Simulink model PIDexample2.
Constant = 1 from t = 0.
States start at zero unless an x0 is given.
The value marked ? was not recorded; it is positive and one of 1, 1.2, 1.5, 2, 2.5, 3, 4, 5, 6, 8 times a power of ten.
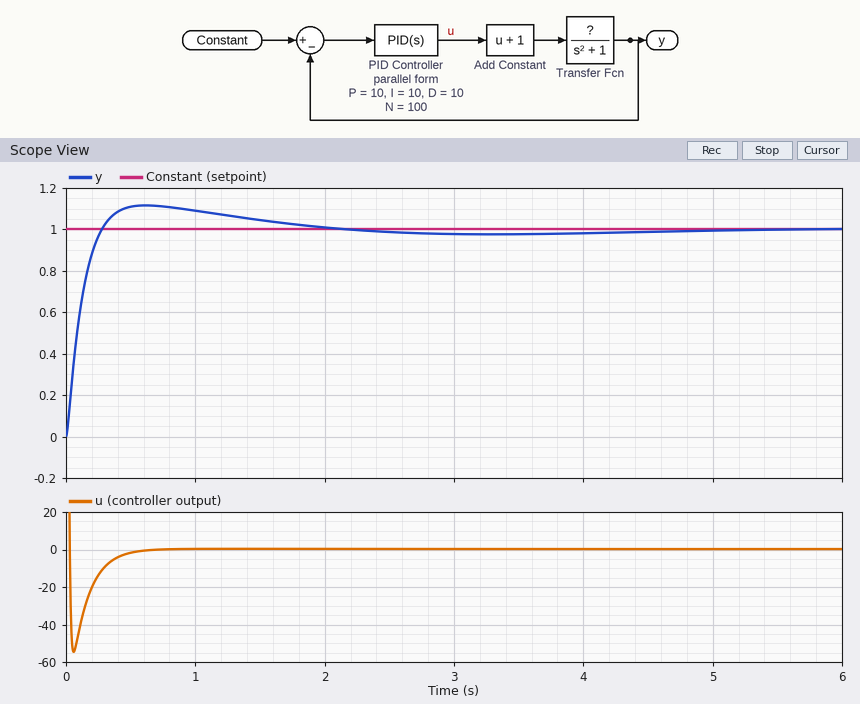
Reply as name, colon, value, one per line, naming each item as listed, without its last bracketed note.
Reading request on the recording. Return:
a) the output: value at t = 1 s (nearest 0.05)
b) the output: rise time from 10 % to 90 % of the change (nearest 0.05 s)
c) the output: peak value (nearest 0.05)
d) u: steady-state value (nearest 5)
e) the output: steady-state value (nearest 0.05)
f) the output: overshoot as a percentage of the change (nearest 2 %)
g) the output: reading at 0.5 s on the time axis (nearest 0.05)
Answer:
the output: value at t = 1 s: 1.10
the output: rise time from 10 % to 90 % of the change: 0.20 s
the output: peak value: 1.10
u: steady-state value: 0
the output: steady-state value: 1.00
the output: overshoot as a percentage of the change: 12 %
the output: reading at 0.5 s on the time axis: 1.10
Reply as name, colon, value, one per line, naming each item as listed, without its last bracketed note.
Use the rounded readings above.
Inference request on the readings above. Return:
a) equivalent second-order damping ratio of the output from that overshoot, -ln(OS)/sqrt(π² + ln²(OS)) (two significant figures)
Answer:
equivalent second-order damping ratio of the output from that overshoot, -ln(OS)/sqrt(π² + ln²(OS)): 0.56
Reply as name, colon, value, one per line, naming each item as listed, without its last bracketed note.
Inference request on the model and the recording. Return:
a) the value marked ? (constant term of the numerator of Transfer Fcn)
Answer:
the value marked ?: 0.8
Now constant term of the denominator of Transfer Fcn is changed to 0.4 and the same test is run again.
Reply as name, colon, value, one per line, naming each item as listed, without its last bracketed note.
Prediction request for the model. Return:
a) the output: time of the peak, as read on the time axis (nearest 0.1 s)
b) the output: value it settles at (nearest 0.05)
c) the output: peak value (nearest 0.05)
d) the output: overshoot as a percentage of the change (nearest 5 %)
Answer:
the output: time of the peak, as read on the time axis: 0.7 s
the output: value it settles at: 1.00
the output: peak value: 1.15
the output: overshoot as a percentage of the change: 15 %
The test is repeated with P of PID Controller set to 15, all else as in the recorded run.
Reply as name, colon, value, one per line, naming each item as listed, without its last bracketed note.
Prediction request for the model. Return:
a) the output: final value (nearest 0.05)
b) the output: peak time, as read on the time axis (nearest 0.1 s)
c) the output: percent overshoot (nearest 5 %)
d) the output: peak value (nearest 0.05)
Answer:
the output: final value: 1.00
the output: peak time, as read on the time axis: 0.5 s
the output: percent overshoot: 15 %
the output: peak value: 1.15
